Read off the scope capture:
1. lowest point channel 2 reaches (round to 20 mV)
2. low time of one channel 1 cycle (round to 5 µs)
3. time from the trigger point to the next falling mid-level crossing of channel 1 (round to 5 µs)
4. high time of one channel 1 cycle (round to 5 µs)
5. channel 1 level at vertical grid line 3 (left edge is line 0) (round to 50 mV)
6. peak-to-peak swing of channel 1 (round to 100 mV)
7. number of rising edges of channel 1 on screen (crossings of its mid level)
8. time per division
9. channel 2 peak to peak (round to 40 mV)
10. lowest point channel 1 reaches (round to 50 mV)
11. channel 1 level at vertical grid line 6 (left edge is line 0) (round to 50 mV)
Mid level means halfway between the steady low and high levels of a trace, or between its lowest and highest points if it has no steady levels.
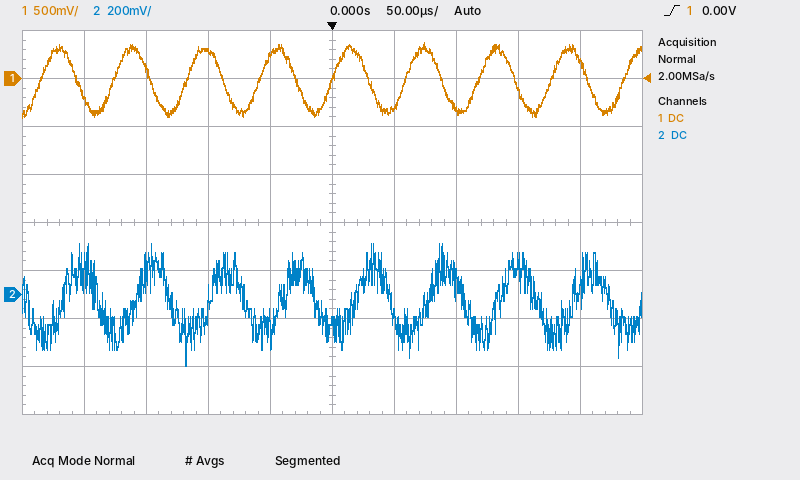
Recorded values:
-300 mV
30 µs
30 µs
30 µs
300 mV
800 mV
9
50 µs
520 mV
-400 mV
-300 mV
